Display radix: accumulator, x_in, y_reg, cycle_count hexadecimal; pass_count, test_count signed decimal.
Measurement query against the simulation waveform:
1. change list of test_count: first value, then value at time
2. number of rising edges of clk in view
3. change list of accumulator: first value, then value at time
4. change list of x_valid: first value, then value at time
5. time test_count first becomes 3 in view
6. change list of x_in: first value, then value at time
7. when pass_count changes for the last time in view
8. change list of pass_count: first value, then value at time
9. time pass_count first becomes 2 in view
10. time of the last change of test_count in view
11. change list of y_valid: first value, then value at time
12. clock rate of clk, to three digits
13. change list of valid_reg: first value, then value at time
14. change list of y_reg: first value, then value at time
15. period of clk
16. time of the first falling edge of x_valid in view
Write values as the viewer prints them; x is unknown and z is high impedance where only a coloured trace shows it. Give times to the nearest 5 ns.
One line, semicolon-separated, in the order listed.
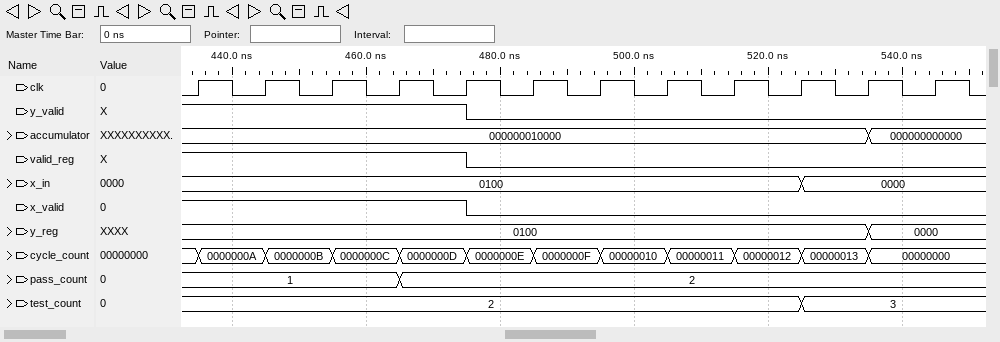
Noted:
2, 3 at 525 ns; 12; 000000010000, 000000000000 at 535 ns; 1, 0 at 475 ns; 525 ns; 0100, 0000 at 525 ns; 465 ns; 1, 2 at 465 ns; 465 ns; 525 ns; 1, 0 at 475 ns; 100 MHz; 1, 0 at 475 ns; 0100, 0000 at 535 ns; 10 ns; 475 ns
